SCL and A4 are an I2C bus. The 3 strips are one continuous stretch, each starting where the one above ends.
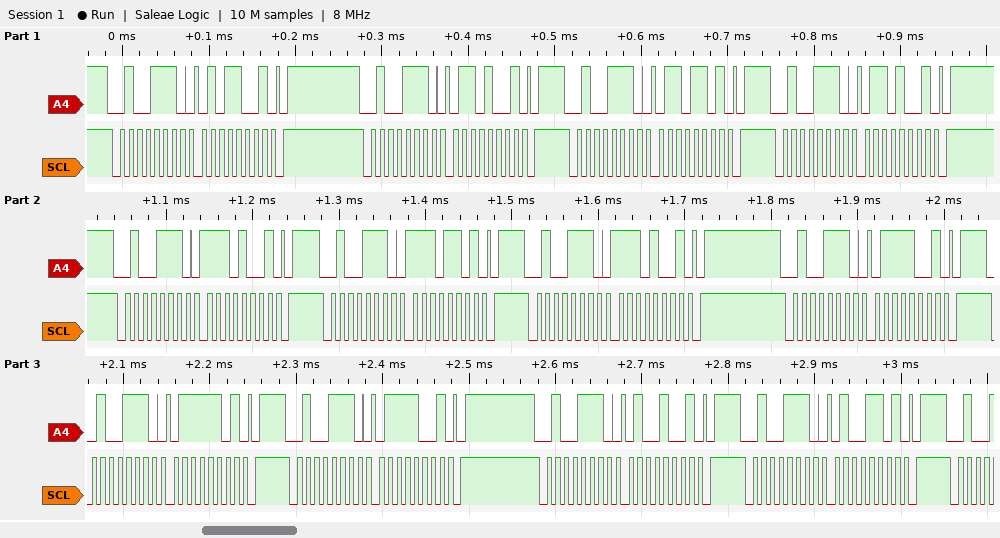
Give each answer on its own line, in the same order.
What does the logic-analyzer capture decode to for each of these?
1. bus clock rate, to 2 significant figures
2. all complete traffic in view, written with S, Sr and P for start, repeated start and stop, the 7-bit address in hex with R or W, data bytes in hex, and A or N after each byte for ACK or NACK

100 kHz
S 27W A 59 A P S 27W A 69 A P S 27W A 6D A P S 27W A 69 A P S 27W A E9 A P S 27W A ED A P S 27W A E9 A P S 27W A 79 A P S 27W A 7D A P S 27W A 79 A P S 27W A 49 A P S 27W A 4D A P
